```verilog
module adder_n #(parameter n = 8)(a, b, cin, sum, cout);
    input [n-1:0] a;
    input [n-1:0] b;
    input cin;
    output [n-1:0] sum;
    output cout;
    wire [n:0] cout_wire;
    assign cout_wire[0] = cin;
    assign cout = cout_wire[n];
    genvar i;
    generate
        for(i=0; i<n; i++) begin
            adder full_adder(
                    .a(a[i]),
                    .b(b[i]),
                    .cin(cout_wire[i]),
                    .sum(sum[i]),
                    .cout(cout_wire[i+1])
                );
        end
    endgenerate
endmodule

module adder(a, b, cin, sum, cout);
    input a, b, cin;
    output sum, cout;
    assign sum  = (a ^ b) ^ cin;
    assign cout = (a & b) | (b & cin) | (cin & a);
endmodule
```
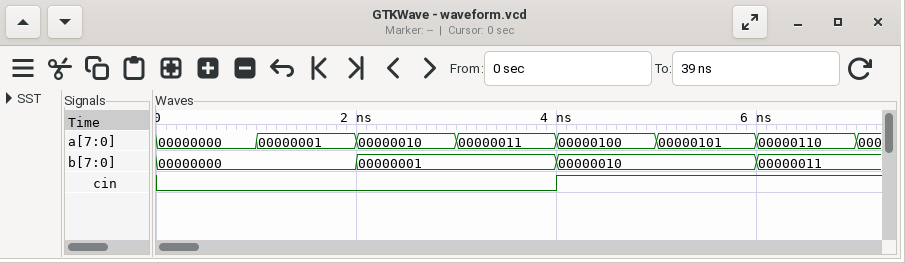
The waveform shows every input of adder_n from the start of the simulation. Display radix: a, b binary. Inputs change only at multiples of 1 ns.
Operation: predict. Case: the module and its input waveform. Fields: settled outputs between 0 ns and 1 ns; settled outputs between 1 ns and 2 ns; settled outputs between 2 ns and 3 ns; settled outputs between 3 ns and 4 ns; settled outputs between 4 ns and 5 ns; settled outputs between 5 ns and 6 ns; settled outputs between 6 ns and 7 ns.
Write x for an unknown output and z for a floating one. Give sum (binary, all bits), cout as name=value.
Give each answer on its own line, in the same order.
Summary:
sum=00000000, cout=0
sum=00000001, cout=0
sum=00000011, cout=0
sum=00000100, cout=0
sum=00000111, cout=0
sum=00001000, cout=0
sum=00001010, cout=0
